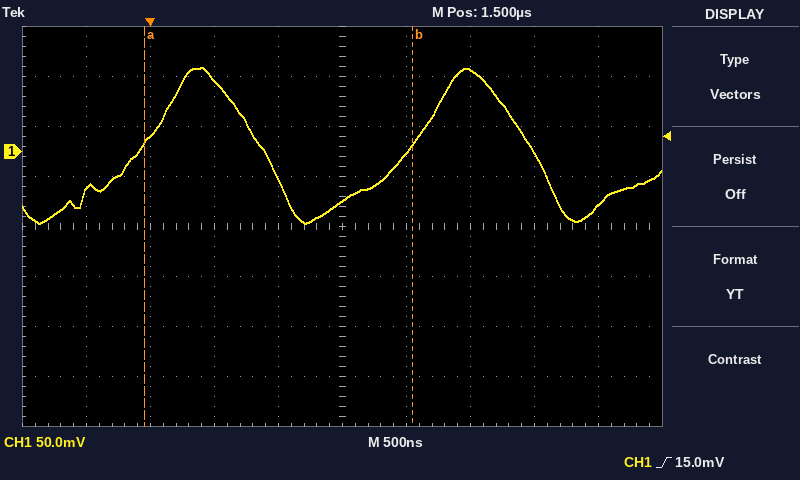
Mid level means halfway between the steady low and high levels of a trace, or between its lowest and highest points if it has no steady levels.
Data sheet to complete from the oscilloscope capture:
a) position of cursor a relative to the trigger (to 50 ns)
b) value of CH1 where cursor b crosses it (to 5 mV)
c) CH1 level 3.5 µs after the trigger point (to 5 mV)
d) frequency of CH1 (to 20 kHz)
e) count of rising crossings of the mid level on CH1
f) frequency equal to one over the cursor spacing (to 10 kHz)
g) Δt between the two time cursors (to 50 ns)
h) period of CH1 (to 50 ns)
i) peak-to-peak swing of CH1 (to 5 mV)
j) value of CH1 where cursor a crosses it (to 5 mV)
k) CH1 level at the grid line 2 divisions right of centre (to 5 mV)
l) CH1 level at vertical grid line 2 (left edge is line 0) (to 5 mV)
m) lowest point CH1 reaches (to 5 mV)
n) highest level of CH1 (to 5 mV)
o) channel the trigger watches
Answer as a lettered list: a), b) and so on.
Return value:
a) -50 ns
b) 5 mV
c) -55 mV
d) 480 kHz
e) 2
f) 480 kHz
g) 2.10 µs
h) 2.10 µs
i) 155 mV
j) 10 mV
k) 80 mV
l) 15 mV
m) -70 mV
n) 85 mV
o) CH1
